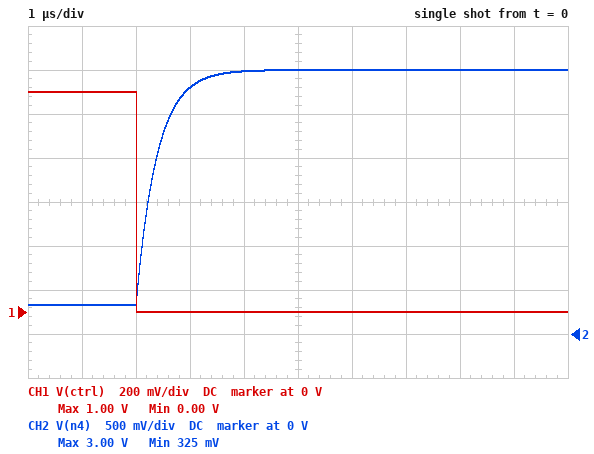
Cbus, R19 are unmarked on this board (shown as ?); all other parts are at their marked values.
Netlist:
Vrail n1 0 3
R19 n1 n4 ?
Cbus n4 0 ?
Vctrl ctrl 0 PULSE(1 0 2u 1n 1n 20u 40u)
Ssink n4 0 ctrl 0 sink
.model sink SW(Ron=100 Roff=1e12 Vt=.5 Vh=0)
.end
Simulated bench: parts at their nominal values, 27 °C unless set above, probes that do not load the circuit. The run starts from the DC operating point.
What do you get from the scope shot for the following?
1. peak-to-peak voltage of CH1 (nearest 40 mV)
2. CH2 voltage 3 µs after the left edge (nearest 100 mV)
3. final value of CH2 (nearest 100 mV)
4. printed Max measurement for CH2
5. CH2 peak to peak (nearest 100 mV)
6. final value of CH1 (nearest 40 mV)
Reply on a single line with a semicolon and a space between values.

1.00 V; 2.8 V; 3.0 V; 3.00 V; 2.7 V; 0 V
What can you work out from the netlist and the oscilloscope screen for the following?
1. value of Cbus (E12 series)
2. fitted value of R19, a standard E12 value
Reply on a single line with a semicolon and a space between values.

470 pF; 820 Ω
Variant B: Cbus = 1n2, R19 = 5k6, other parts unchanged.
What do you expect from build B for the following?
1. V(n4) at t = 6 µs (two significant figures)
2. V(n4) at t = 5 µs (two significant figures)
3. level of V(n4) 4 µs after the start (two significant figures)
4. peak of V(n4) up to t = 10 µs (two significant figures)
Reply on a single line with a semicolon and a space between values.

1.4 V; 1.1 V; 810 mV; 2.1 V
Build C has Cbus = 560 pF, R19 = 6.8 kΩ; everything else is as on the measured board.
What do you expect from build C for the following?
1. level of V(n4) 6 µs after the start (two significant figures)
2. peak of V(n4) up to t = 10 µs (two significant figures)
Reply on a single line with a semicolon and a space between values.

2.0 V; 2.6 V
